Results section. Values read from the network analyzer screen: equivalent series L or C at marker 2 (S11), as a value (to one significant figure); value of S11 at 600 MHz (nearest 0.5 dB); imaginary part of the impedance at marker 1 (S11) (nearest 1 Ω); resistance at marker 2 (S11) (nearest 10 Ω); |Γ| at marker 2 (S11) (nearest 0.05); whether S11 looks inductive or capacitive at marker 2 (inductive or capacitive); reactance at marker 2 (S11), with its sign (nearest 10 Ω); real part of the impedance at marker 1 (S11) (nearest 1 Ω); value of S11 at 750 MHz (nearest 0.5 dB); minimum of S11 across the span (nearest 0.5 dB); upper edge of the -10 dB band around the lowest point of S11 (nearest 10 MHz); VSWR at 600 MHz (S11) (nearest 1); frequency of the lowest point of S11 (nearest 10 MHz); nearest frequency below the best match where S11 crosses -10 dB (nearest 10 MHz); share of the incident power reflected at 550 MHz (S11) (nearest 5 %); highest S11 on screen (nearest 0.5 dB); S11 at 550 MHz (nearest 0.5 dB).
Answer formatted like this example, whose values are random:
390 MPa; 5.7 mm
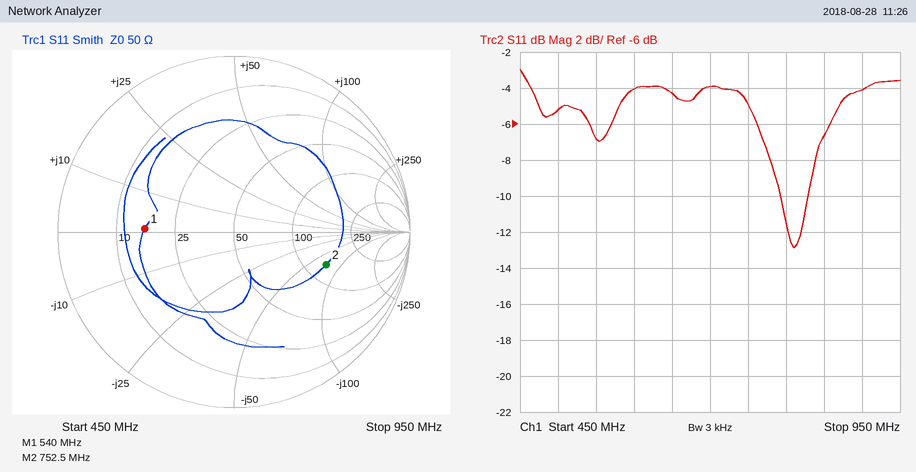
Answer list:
3 pF; -4.0 dB; +1 Ω; 130 Ω; 0.55; capacitive; -70 Ω; 16 Ω; -5.0 dB; -13.0 dB; 830 MHz; 4; 810 MHz; 790 MHz; 20 %; -3.0 dB; -7.0 dB
